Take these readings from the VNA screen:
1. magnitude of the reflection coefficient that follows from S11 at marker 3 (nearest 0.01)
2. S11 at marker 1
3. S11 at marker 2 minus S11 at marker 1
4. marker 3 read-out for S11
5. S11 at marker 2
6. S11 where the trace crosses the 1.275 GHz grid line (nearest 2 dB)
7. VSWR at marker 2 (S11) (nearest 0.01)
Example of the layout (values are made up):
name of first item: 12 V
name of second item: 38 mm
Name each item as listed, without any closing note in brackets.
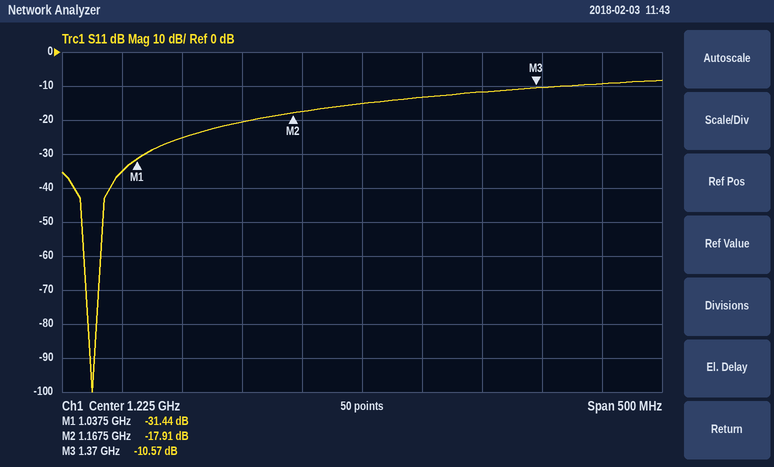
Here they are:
magnitude of the reflection coefficient that follows from S11 at marker 3: 0.30
S11 at marker 1: -31.44 dB
S11 at marker 2 minus S11 at marker 1: 13.53 dB
marker 3 read-out for S11: -10.57 dB
S11 at marker 2: -17.91 dB
S11 where the trace crosses the 1.275 GHz grid line: -14 dB
VSWR at marker 2 (S11): 1.29
